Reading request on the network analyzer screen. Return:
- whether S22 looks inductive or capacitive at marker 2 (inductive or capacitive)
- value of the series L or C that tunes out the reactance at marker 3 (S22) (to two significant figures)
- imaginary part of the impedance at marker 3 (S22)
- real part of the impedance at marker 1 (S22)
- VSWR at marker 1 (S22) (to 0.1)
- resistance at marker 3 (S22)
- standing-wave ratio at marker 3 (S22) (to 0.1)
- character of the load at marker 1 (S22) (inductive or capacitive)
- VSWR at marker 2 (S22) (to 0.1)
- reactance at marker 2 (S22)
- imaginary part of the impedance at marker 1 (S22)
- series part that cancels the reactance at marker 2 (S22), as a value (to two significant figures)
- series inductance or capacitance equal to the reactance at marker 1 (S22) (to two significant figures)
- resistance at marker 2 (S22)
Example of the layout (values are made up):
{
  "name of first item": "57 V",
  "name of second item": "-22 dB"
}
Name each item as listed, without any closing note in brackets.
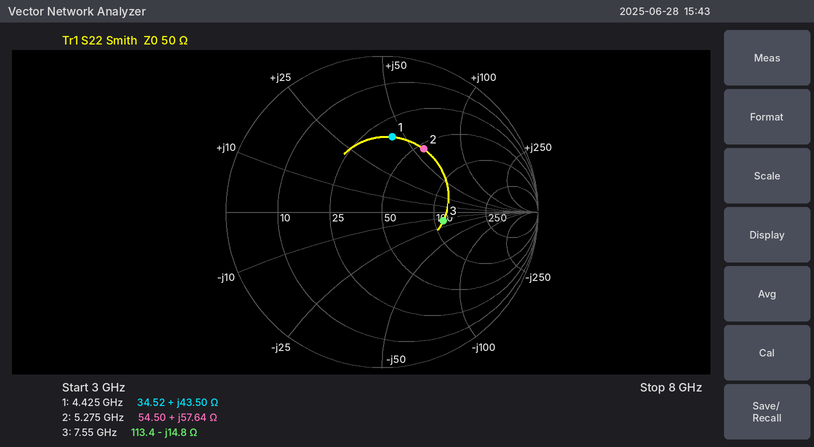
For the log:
{
  "whether S22 looks inductive or capacitive at marker 2": "inductive",
  "value of the series L or C that tunes out the reactance at marker 3 (S22)": "310 pH",
  "imaginary part of the impedance at marker 3": "-14.8 Ω",
  "real part of the impedance at marker 1": "34.52 Ω",
  "VSWR at marker 1 (S22)": "2.9",
  "resistance at marker 3": "113.4 Ω",
  "standing-wave ratio at marker 3 (S22)": "2.3",
  "character of the load at marker 1 (S22)": "inductive",
  "VSWR at marker 2 (S22)": "2.9",
  "reactance at marker 2": "+57.64 Ω",
  "imaginary part of the impedance at marker 1": "+43.50 Ω",
  "series part that cancels the reactance at marker 2 (S22), as a value": "520 fF",
  "series inductance or capacitance equal to the reactance at marker 1 (S22)": "1.6 nH",
  "resistance at marker 2": "54.50 Ω"
}
